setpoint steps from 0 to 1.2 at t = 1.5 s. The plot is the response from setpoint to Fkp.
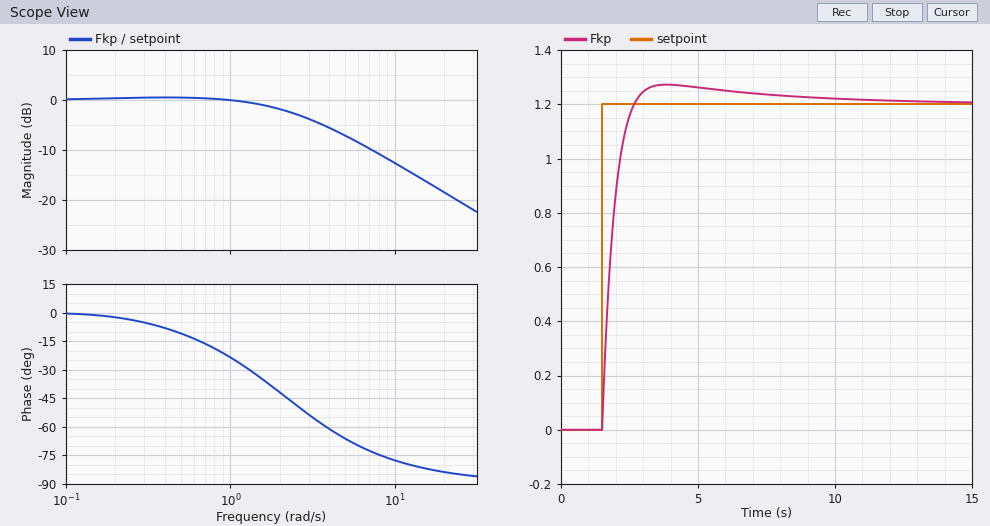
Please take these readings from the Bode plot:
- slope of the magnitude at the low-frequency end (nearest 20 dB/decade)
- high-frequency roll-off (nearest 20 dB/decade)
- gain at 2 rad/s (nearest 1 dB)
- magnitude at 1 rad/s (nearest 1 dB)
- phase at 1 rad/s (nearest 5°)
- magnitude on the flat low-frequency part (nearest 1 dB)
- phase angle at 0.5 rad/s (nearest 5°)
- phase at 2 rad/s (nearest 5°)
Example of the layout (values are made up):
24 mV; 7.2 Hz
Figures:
0 dB/decade; -20 dB/decade; -2 dB; 0 dB; -25°; 0 dB; -10°; -40°
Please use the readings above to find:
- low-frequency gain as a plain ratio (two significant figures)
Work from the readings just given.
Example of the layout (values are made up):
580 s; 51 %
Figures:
1.0
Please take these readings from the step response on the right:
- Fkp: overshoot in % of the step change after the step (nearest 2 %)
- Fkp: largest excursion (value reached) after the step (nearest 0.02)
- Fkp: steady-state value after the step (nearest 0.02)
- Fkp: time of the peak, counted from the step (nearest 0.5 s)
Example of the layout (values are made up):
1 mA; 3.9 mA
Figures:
6 %; 1.28; 1.20; 2.5 s
